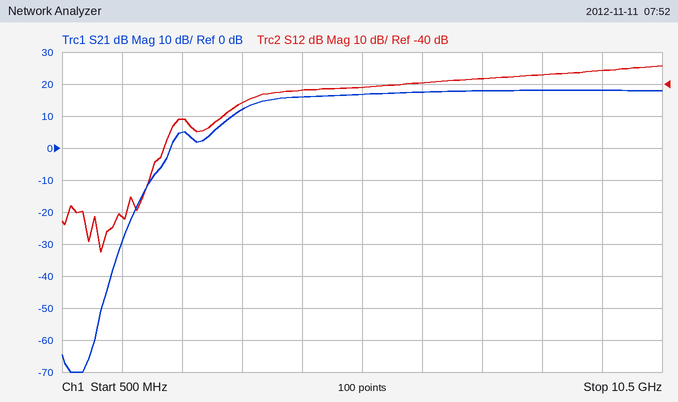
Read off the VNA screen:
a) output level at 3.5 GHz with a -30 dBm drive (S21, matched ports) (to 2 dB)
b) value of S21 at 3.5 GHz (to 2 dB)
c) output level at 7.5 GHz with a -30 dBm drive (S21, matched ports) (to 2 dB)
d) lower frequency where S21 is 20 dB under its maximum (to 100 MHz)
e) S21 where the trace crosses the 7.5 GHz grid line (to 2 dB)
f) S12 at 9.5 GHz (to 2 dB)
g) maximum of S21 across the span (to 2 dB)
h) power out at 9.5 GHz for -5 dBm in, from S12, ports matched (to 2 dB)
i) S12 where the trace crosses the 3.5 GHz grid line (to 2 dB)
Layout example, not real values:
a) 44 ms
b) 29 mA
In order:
a) -18 dBm
b) 12 dB
c) -12 dBm
d) 2.3 GHz
e) 18 dB
f) -36 dB
g) 18 dB
h) -40 dBm
i) -46 dB
